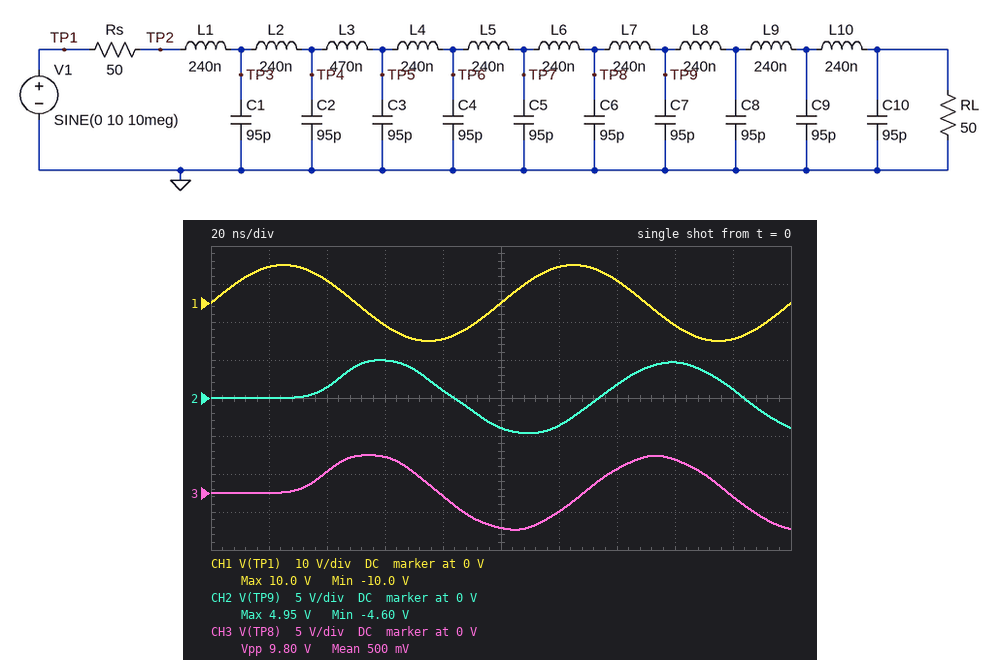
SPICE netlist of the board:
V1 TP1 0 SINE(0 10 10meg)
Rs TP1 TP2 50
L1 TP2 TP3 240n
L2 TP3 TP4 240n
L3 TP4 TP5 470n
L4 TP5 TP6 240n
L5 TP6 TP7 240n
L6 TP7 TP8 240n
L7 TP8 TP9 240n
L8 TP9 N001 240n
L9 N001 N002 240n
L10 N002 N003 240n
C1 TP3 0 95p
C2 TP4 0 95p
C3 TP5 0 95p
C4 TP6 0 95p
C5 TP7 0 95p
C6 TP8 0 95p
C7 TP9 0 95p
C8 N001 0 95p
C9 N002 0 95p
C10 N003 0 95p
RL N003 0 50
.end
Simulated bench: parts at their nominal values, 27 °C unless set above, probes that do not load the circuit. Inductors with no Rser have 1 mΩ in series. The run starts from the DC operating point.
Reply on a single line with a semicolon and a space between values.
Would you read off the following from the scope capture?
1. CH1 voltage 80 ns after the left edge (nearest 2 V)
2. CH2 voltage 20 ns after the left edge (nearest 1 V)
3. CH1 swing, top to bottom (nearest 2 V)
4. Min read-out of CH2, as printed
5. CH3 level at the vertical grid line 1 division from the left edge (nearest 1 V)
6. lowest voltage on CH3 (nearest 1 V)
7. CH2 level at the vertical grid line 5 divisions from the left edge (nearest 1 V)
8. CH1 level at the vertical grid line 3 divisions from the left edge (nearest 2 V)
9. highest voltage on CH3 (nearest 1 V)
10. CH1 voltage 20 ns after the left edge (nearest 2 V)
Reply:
-10 V; 0 V; 20 V; -4.60 V; 0 V; -5 V; -4 V; -6 V; 5 V; 10 V
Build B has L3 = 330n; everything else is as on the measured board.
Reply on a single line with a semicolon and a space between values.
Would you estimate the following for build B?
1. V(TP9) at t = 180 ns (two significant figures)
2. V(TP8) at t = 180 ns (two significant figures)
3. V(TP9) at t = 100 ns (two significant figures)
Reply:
780 mV; -860 mV; -4.2 V
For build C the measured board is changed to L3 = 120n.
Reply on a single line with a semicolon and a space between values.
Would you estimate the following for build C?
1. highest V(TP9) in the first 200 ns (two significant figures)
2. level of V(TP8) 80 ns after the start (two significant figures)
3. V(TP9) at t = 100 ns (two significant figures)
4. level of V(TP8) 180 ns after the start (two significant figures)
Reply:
4.9 V; -1.5 V; -4.4 V; -1.4 V
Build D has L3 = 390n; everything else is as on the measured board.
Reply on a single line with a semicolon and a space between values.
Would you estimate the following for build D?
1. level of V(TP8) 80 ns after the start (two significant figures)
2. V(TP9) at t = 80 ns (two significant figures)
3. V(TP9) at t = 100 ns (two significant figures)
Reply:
-630 mV; 780 mV; -4.1 V
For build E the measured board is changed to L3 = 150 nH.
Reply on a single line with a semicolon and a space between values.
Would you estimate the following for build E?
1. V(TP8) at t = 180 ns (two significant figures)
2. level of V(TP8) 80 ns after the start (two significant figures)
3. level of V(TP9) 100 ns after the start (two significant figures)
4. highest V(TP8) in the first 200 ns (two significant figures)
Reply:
-1.3 V; -1.4 V; -4.4 V; 4.9 V
